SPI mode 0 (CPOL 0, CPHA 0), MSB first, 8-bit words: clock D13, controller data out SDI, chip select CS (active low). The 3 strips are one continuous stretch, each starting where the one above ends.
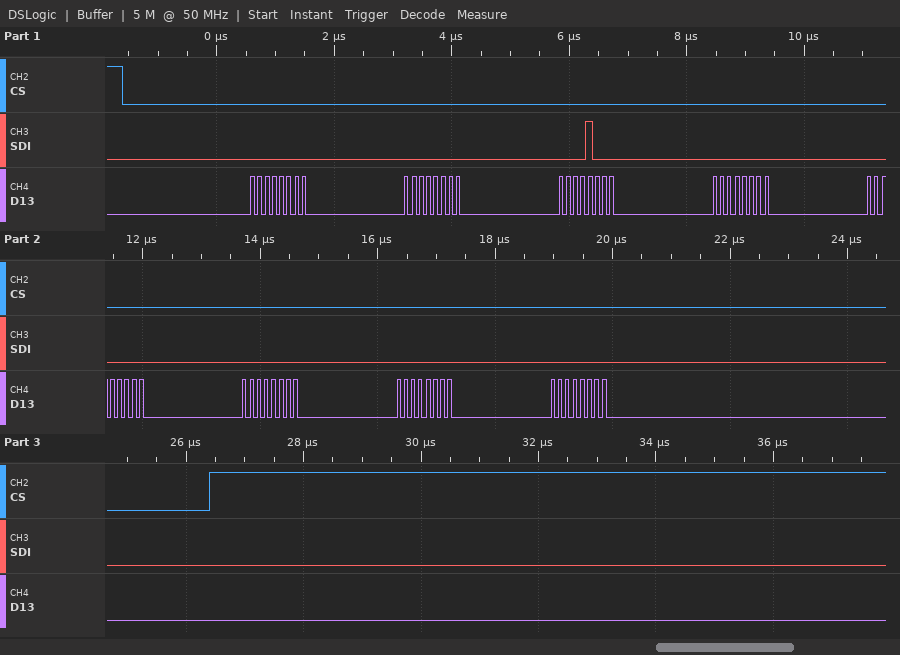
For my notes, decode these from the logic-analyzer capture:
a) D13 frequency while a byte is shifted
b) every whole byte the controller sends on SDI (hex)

8 MHz
00 00 08 00 00 00 00 00
